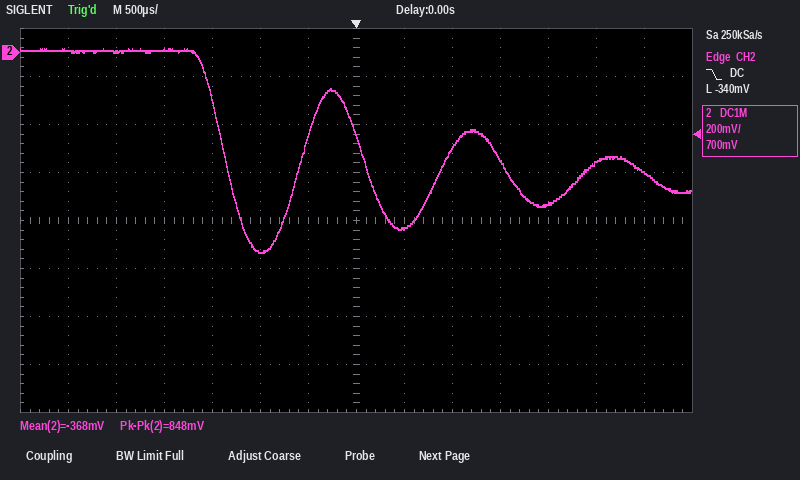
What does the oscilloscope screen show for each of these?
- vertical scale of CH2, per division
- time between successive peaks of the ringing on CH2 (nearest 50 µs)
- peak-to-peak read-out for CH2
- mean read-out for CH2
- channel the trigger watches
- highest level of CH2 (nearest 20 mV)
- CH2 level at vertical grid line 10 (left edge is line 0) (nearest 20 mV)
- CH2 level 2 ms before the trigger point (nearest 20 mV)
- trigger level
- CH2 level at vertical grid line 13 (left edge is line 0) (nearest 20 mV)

200 mV
1.50 ms
848 mV
-368 mV
CH2
20 mV
-440 mV
20 mV
-340 mV
-500 mV
